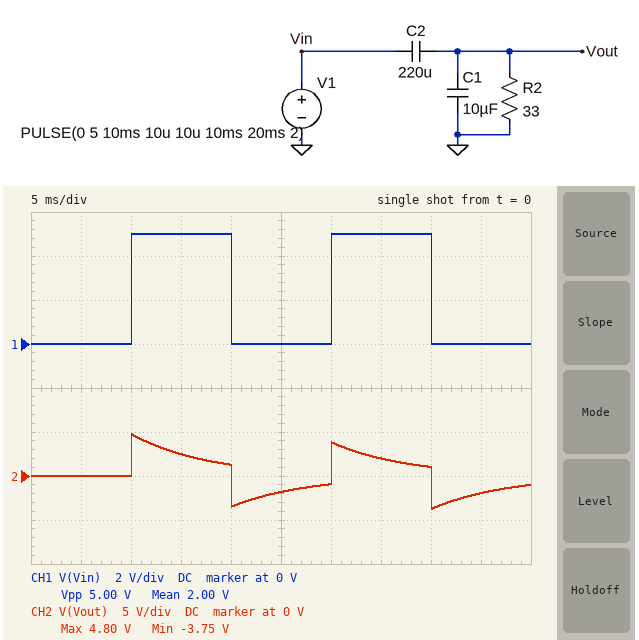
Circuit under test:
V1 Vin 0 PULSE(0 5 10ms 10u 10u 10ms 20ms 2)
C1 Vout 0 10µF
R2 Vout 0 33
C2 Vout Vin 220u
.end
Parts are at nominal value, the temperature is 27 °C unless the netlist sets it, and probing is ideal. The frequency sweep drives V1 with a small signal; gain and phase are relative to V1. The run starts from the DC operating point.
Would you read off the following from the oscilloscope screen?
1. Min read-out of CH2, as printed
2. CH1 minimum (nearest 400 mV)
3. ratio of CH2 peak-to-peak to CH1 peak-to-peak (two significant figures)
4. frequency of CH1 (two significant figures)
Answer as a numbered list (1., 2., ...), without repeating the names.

1. -3.75 V
2. 0 V
3. 1.7
4. 50 Hz
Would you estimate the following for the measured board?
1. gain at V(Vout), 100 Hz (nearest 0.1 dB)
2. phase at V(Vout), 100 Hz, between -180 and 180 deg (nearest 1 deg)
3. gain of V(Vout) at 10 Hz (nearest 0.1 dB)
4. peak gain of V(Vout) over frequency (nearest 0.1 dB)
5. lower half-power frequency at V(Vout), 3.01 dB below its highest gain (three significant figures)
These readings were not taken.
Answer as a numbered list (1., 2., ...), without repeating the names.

1. -0.6 dB
2. 12 deg
3. -7.7 dB
4. -0.4 dB
5. 21.0 Hz
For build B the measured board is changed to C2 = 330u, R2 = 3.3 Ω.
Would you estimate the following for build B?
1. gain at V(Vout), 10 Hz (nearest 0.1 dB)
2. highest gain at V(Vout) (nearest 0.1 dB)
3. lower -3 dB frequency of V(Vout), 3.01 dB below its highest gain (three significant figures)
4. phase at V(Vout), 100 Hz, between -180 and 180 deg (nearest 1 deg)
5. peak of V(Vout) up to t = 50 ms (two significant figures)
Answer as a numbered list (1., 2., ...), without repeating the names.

1. -23.3 dB
2. -0.3 dB
3. 142 Hz
4. 55 deg
5. 4.8 V
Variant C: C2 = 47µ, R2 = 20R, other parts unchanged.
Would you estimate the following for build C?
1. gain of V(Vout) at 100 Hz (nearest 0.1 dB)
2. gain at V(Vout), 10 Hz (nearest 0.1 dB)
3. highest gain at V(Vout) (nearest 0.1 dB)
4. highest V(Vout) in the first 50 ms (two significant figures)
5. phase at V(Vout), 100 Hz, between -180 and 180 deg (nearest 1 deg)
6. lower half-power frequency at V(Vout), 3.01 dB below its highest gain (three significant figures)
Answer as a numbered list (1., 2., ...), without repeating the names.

1. -6.4 dB
2. -24.6 dB
3. -1.7 dB
4. 4.1 V
5. 54 deg
6. 140 Hz
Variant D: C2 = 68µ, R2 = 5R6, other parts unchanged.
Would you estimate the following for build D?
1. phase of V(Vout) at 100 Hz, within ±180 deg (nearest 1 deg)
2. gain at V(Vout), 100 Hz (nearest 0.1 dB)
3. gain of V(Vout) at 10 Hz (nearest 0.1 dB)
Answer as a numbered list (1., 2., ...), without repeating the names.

1. 75 deg
2. -12.7 dB
3. -32.4 dB
